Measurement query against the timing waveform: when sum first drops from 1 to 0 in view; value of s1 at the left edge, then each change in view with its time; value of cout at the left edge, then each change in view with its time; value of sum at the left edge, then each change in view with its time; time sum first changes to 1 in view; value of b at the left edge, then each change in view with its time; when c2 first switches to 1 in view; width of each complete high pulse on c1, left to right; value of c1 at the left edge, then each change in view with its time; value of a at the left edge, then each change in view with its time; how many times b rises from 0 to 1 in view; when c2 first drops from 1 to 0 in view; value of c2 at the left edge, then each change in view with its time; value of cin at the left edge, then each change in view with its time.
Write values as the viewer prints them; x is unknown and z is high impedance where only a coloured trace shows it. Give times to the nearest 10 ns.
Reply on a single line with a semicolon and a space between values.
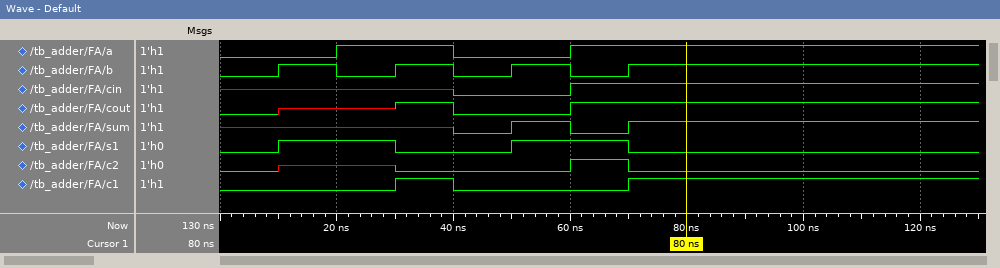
60 ns; 0, 1 at 10 ns, 0 at 30 ns, 1 at 50 ns, 0 at 70 ns; 0, x at 10 ns, 1 at 30 ns, 0 at 40 ns, 1 at 60 ns; x, 0 at 40 ns, 1 at 50 ns, 0 at 60 ns, 1 at 70 ns; 50 ns; 0, 1 at 10 ns, 0 at 20 ns, 1 at 30 ns, 0 at 40 ns, 1 at 50 ns, 0 at 60 ns, 1 at 70 ns; 60 ns; 10 ns; 0, 1 at 30 ns, 0 at 40 ns, 1 at 70 ns; 0, 1 at 20 ns, 0 at 40 ns, 1 at 60 ns; 4; 70 ns; 0, x at 10 ns, 0 at 30 ns, 1 at 60 ns, 0 at 70 ns; x, 0 at 40 ns, 1 at 60 ns
